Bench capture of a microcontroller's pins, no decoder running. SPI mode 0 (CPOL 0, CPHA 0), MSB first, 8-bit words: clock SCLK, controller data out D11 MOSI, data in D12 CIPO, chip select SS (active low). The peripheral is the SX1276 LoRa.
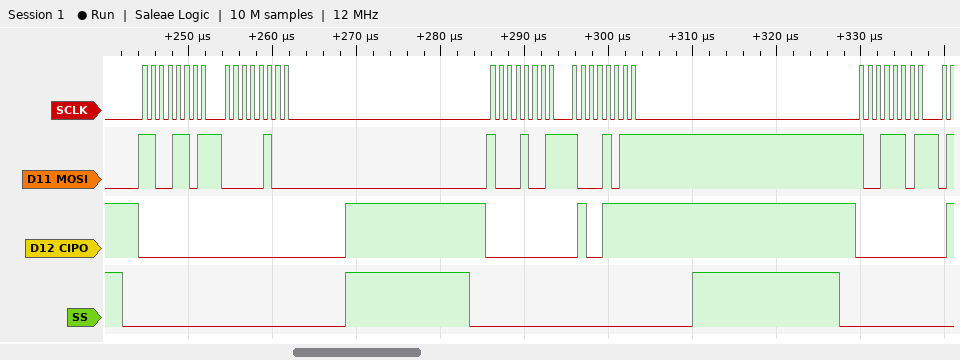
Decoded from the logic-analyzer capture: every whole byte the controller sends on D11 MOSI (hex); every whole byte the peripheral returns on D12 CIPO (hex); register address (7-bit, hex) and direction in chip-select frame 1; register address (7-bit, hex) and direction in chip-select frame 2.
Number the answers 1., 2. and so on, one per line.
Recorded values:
1. CD 04 89 8B 9D
2. 00 00 00 4F 00
3. 0x4D write
4. 0x09 write
